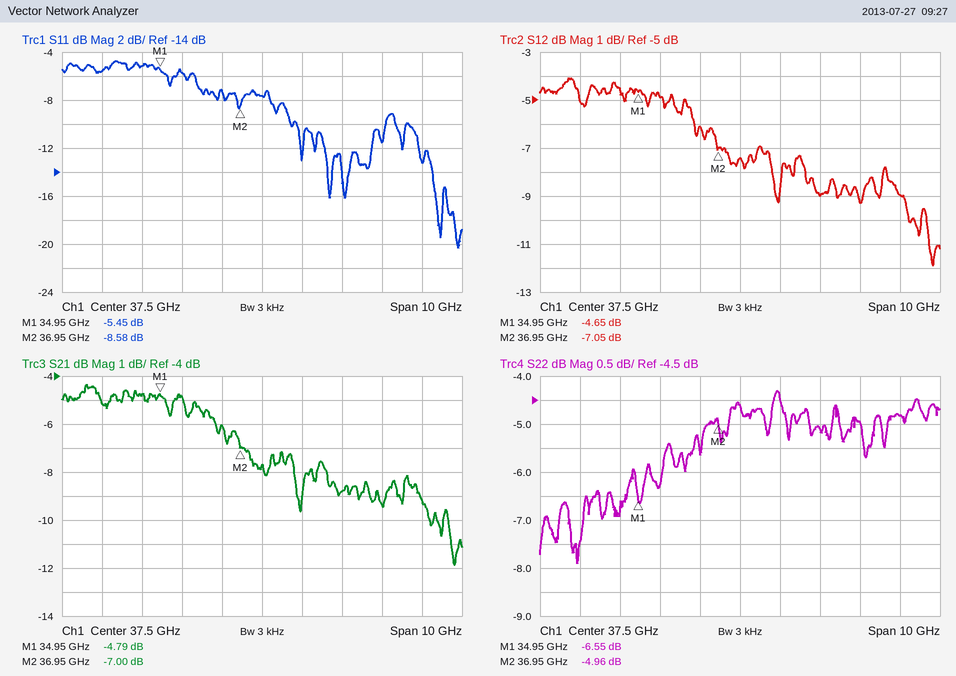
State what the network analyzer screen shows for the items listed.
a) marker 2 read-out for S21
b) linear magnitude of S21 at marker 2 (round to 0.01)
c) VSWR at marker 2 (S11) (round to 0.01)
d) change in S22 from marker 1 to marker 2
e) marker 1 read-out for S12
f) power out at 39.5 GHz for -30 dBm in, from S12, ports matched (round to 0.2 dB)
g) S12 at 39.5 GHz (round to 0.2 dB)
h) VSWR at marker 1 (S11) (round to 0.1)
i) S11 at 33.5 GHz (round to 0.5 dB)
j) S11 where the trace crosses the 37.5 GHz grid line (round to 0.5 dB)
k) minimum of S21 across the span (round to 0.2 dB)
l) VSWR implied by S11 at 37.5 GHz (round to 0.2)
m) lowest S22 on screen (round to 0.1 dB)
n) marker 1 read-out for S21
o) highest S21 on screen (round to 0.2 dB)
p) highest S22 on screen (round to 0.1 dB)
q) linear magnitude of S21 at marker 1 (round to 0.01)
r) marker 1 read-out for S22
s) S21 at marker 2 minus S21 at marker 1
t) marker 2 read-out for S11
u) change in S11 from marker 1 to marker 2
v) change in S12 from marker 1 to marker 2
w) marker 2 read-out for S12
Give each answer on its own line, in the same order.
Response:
-7.00 dB
0.45
2.19
1.59 dB
-4.65 dB
-39.0 dBm
-9.0 dB
3.3
-5.5 dB
-7.5 dB
-11.8 dB
2.4
-7.9 dB
-4.79 dB
-4.4 dB
-4.3 dB
0.58
-6.55 dB
-2.21 dB
-8.58 dB
-3.13 dB
-2.40 dB
-7.05 dB
